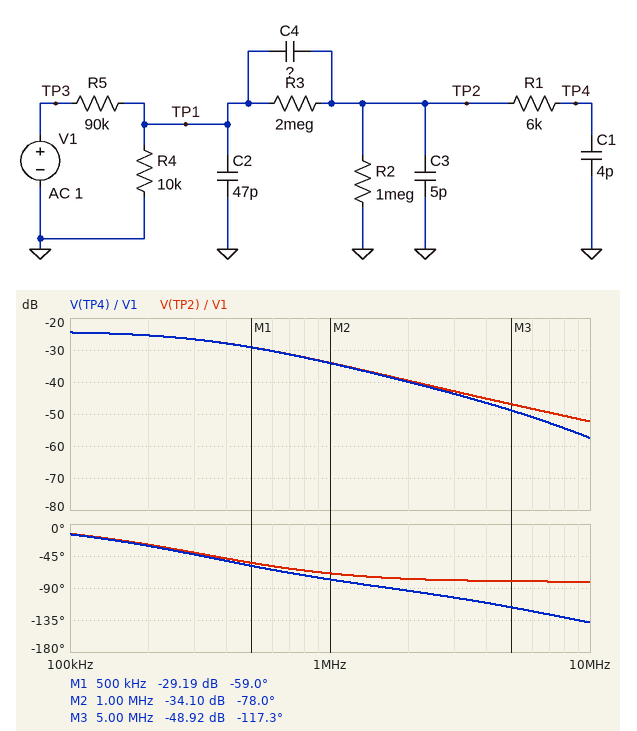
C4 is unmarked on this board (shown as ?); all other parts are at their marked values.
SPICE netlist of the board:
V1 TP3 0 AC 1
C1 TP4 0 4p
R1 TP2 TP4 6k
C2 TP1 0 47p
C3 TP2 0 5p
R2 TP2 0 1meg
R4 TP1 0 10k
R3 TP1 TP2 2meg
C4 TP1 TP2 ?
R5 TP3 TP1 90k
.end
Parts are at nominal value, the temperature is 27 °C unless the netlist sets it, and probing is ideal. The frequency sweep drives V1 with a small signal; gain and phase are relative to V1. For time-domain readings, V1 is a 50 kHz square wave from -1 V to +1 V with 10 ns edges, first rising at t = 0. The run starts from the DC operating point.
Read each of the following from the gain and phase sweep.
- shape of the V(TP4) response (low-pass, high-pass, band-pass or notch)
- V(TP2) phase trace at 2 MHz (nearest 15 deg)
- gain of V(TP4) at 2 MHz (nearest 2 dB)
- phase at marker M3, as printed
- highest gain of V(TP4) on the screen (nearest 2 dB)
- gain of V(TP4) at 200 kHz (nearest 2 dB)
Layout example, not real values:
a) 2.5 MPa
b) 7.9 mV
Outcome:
a) low-pass
b) -75 deg
c) -40 dB
d) -117.3 deg
e) -24 dB
f) -26 dB
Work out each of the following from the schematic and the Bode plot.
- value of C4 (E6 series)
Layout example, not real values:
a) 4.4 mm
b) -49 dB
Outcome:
a) 15 pF
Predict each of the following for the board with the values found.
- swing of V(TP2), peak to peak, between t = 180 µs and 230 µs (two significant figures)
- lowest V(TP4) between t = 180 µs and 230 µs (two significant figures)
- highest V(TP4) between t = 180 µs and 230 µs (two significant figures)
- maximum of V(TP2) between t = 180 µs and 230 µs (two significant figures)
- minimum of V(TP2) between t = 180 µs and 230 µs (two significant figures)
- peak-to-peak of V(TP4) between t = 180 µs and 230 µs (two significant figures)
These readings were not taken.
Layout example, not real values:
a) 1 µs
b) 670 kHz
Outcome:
a) 130 mV
b) -66 mV
c) 66 mV
d) 66 mV
e) -66 mV
f) 130 mV
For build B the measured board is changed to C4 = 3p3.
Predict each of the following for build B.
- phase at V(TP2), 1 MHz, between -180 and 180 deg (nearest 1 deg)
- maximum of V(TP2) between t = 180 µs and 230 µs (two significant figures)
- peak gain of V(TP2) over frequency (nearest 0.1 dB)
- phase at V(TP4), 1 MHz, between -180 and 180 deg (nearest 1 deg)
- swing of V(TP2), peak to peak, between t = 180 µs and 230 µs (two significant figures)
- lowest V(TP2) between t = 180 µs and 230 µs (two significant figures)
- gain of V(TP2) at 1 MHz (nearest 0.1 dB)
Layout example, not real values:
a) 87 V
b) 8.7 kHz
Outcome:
a) -68 deg
b) 30 mV
c) -29.6 dB
d) -76 deg
e) 60 mV
f) -30 mV
g) -40.8 dB
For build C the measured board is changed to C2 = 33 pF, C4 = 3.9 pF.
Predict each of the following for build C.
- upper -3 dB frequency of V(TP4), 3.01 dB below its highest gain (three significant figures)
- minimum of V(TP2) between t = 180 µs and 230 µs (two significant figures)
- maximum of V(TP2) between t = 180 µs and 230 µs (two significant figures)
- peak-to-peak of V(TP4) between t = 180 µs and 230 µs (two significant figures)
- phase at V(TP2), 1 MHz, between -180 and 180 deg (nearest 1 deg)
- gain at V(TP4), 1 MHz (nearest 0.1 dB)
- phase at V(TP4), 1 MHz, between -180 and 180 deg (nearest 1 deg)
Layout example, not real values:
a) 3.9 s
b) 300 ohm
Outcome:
a) 397 kHz
b) -32 mV
c) 32 mV
d) 63 mV
e) -61 deg
f) -37.5 dB
g) -70 deg
